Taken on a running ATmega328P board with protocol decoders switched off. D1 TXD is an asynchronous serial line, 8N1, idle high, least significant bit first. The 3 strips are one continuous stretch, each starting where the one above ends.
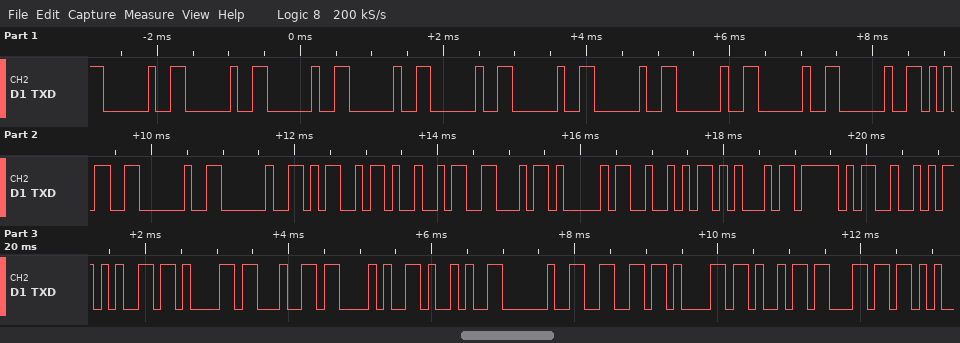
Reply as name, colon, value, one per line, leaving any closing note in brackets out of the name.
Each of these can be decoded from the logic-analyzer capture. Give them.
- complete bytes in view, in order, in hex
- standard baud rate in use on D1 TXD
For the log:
complete bytes in view, in order, in hex: 0x20 0x20 0x20 0x20 0x20 0x20 0x20 0x20 0x20 0x20 0x35 0x20 0x20 0x4D 0x49 0x46 0x41 0x52 0x45 0x5F 0x52 0x65 0x61 0x64 0x28 0x29 0x20 0x66 0x61 0x69 0x6C
standard baud rate in use on D1 TXD: 9600 baud
